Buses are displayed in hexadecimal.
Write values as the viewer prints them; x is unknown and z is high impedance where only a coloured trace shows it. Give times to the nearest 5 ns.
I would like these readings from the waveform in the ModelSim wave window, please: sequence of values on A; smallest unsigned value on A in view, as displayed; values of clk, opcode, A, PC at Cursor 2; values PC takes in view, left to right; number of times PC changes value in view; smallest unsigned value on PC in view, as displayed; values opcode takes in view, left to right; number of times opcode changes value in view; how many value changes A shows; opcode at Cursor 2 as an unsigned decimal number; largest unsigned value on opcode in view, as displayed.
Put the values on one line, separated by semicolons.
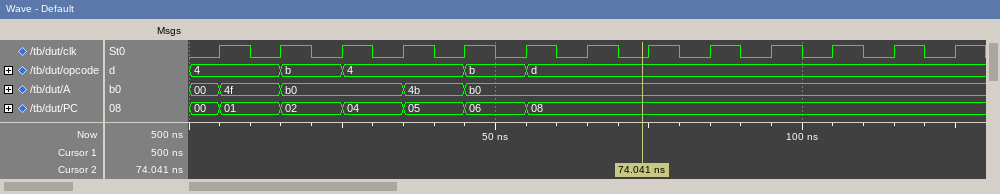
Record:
00, 4f, b0, 4b, b0; 00; clk=0, opcode=d, A=b0, PC=08; 00, 01, 02, 04, 05, 06, 08; 6; 00; 4, b, 4, b, d; 4; 4; 13; d
